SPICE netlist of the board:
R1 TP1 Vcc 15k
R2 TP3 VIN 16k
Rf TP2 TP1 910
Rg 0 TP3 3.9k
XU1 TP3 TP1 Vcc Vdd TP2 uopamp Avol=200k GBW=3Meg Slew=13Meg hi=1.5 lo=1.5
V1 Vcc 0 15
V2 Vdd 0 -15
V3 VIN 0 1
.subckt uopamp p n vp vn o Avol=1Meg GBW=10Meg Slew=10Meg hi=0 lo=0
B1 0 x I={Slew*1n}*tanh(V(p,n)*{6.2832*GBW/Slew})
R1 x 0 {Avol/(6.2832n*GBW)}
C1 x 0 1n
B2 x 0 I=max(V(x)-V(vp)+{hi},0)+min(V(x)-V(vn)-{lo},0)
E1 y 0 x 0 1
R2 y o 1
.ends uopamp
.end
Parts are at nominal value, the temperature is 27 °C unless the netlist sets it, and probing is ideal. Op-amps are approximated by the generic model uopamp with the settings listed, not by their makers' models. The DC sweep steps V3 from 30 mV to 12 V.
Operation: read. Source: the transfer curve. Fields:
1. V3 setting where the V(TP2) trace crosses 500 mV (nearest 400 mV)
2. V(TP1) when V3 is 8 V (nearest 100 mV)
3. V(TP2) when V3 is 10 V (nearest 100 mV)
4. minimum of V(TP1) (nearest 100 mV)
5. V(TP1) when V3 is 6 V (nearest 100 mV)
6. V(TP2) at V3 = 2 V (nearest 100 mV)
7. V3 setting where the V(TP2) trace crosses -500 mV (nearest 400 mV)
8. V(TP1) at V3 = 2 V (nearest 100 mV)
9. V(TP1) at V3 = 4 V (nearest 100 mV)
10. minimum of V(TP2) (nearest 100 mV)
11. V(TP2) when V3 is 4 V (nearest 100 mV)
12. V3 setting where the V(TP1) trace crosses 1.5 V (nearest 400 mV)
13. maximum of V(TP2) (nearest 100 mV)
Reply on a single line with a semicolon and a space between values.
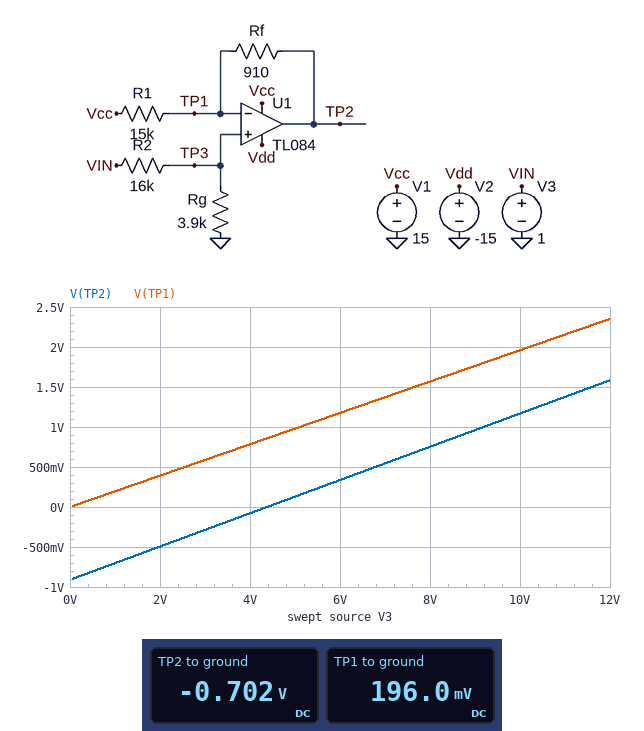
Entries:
6.8 V; 1.6 V; 1.2 V; 0 V; 1.2 V; -500 mV; 2.0 V; 400 mV; 800 mV; -900 mV; -100 mV; 7.6 V; 1.6 V
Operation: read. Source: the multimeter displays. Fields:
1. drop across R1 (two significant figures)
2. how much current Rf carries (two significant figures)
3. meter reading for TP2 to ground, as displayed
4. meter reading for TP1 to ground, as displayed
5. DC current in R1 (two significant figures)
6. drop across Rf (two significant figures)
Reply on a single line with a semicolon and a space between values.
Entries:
15 V; 990 µA; -0.702 V; 196.0 mV; 990 µA; 900 mV
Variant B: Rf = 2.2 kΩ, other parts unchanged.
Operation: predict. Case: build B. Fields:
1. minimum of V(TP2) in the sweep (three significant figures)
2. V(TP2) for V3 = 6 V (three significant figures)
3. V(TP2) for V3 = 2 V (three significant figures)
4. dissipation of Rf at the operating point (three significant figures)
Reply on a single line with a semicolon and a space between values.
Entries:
-2.19 V; -852 mV; -1.75 V; 2.14 mW
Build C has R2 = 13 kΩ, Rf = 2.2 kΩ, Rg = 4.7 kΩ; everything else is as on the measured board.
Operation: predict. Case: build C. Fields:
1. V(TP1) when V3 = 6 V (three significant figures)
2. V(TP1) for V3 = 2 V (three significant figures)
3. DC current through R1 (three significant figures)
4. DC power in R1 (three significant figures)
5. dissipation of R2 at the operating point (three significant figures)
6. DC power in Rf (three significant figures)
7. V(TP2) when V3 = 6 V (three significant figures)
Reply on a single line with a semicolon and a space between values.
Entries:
1.59 V; 531 mV; 982 µA; 14.5 mW; 41.5 µW; 2.12 mW; -373 mV
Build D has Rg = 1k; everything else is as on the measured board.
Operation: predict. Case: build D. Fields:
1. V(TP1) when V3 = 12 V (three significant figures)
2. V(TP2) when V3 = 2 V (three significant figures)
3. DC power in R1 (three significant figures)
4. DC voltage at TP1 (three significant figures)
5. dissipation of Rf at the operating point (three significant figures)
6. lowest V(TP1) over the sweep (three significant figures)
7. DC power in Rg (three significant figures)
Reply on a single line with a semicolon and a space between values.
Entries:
706 mV; -785 mV; 14.9 mW; 58.8 mV; 903 µW; 1.77 mV; 3.46 µW
